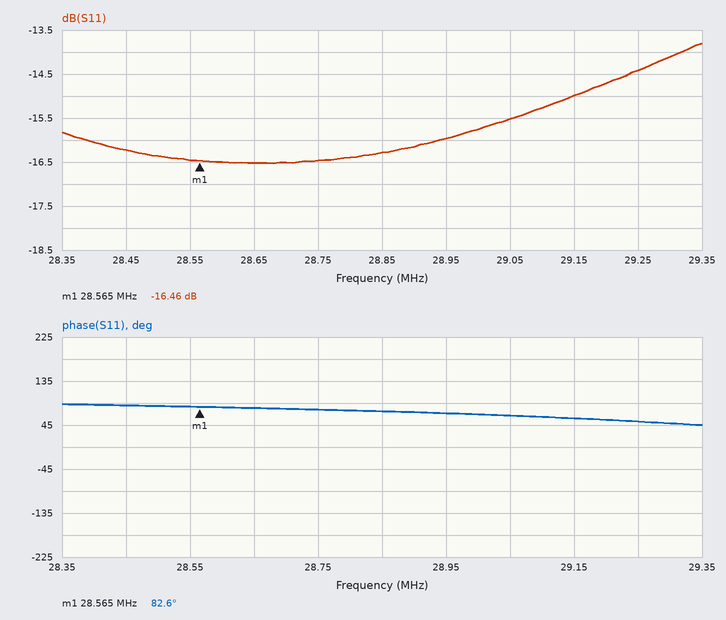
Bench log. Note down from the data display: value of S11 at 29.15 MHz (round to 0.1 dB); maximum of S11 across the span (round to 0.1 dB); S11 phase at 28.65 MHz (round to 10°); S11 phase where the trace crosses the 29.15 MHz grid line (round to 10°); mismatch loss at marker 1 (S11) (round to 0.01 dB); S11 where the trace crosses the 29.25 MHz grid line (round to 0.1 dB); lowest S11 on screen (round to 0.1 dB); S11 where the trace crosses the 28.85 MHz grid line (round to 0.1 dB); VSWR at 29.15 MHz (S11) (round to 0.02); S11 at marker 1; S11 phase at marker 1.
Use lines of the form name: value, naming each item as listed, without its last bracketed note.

value of S11 at 29.15 MHz: -15.0 dB
maximum of S11 across the span: -13.8 dB
S11 phase at 28.65 MHz: 80°
S11 phase where the trace crosses the 29.15 MHz grid line: 60°
mismatch loss at marker 1 (S11): 0.10 dB
S11 where the trace crosses the 29.25 MHz grid line: -14.4 dB
lowest S11 on screen: -16.5 dB
S11 where the trace crosses the 28.85 MHz grid line: -16.3 dB
VSWR at 29.15 MHz (S11): 1.44
S11 at marker 1: -16.46 dB
S11 phase at marker 1: 82.6°
